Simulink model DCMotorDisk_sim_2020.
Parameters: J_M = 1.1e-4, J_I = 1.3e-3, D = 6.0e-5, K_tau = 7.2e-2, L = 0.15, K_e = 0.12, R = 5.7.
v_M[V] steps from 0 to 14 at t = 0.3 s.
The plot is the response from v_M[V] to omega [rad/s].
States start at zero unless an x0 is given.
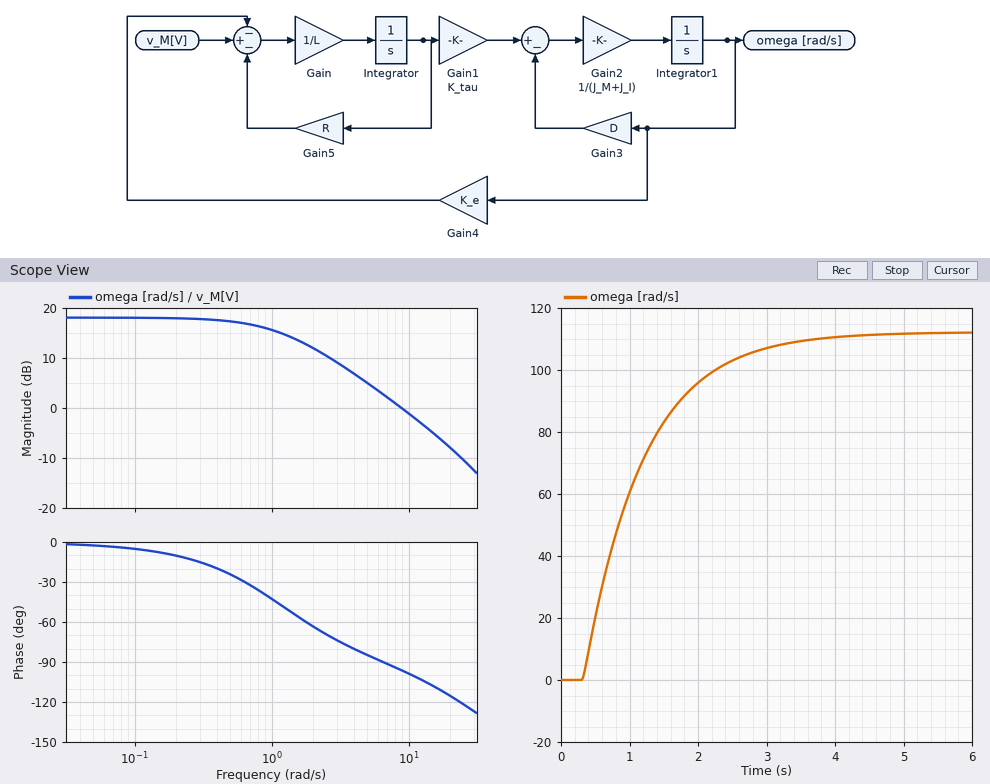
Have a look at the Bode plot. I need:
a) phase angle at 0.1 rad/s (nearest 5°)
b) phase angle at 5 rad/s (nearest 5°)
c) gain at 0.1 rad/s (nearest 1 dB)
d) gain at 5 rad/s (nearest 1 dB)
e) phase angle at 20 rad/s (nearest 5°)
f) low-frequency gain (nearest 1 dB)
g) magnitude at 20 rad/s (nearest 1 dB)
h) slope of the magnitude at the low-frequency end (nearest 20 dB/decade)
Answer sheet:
-5°
-85°
18 dB
5 dB
-115°
18 dB
-8 dB
0 dB/decade
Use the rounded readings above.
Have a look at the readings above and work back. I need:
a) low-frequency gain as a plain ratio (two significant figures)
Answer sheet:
7.9
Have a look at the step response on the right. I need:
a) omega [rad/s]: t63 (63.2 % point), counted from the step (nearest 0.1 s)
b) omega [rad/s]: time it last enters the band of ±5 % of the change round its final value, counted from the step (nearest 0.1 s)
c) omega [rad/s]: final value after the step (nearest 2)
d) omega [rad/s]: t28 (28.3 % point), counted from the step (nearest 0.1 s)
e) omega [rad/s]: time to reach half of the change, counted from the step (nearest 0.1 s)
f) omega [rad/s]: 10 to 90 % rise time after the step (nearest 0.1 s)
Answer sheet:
0.9 s
2.6 s
112
0.3 s
0.6 s
1.9 s
